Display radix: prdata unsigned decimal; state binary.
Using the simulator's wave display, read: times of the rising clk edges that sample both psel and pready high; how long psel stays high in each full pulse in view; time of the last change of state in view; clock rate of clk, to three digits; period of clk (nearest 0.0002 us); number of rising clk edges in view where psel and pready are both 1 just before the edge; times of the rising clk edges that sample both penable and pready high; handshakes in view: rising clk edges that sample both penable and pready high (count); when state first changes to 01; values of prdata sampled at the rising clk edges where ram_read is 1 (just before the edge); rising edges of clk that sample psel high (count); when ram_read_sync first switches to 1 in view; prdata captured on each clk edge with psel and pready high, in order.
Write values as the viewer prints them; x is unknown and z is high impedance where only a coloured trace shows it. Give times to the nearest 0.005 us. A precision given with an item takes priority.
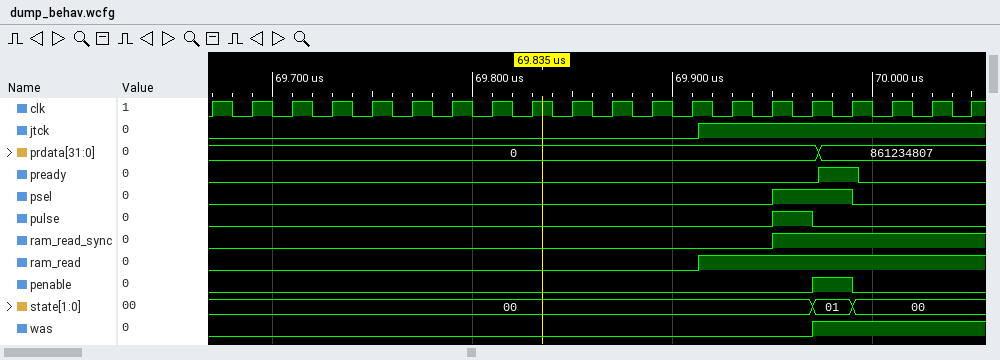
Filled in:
69.99 us
0.04 us
69.99 us
50.0 MHz
0.02 us
1
69.99 us
1
69.97 us
0, 0, 0, 861234807, 861234807, 861234807, 861234807
2
69.95 us
861234807
